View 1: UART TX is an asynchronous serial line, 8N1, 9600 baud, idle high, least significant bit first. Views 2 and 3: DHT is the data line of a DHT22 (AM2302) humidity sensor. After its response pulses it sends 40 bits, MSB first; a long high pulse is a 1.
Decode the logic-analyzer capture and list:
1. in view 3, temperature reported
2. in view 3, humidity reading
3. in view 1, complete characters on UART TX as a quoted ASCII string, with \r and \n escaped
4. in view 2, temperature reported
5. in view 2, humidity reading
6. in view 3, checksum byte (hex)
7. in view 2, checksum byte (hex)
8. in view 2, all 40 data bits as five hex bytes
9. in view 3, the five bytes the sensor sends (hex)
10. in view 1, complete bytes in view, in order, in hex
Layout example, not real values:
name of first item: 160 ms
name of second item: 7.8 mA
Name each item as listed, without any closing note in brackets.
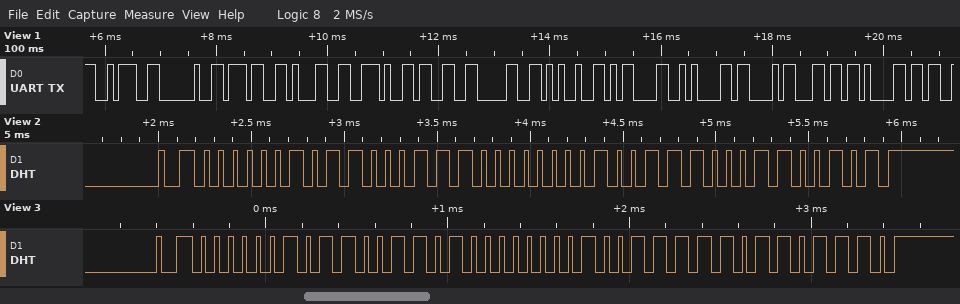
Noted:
in view 3, temperature reported: 15.9 °C
in view 3, humidity reading: 71.7 %
in view 1, complete characters on UART TX as a quoted ASCII string, with \r and \n escaped: ": 71.30%\r\nCla"
in view 2, temperature reported: 15.6 °C
in view 2, humidity reading: 71.1 %
in view 3, checksum byte: 0x6E
in view 2, checksum byte: 0x65
in view 2, all 40 data bits as five hex bytes: 02 C7 00 9C 65
in view 3, the five bytes the sensor sends: 02 CD 00 9F 6E
in view 1, complete bytes in view, in order, in hex: 3A 20 37 31 2E 33 30 25 0D 0A 43 6C 61
